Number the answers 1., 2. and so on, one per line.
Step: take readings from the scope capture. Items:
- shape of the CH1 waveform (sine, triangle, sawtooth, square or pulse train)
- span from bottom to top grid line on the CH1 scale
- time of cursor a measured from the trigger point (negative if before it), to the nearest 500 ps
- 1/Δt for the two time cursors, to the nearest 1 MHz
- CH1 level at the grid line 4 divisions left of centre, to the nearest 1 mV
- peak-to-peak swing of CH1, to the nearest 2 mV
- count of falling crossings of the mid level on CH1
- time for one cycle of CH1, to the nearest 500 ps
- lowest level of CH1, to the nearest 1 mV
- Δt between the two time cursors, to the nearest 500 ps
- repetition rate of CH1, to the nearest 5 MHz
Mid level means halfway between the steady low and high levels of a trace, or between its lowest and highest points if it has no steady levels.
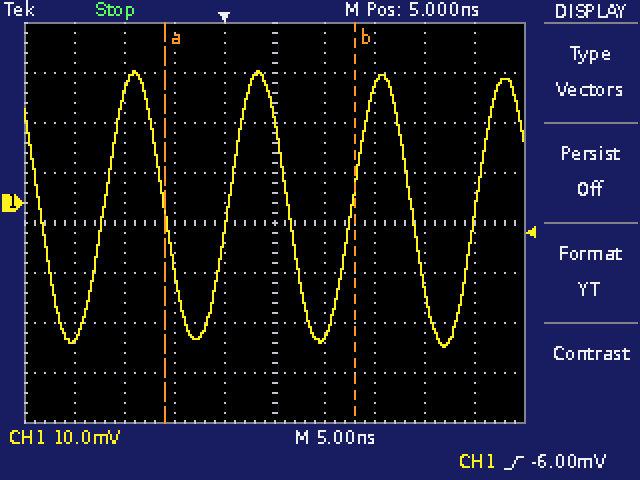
1. sine
2. 80 mV
3. -6.0 ns
4. 53 MHz
5. -27 mV
6. 56 mV
7. 4
8. 12.5 ns
9. -29 mV
10. 19.0 ns
11. 80 MHz
